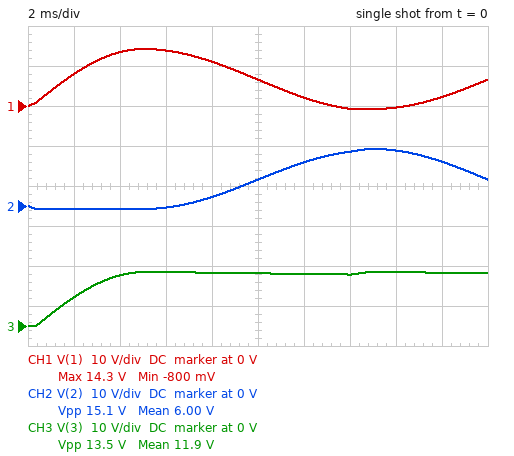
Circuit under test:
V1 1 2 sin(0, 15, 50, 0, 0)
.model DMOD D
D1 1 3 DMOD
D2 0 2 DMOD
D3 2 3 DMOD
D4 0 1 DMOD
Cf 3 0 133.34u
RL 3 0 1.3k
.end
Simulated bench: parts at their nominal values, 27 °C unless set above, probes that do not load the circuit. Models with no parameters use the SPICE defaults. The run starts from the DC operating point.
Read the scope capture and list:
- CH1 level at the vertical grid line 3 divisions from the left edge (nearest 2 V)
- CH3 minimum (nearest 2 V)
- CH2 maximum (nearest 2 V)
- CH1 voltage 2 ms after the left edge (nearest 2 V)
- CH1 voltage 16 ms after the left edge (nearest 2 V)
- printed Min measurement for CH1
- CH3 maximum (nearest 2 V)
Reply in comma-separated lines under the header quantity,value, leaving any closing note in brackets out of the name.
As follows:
quantity,value
CH1 level at the vertical grid line 3 divisions from the left edge,14 V
CH3 minimum,0 V
CH2 maximum,14 V
CH1 voltage 2 ms after the left edge,8 V
CH1 voltage 16 ms after the left edge,0 V
printed Min measurement for CH1,-800 mV
CH3 maximum,14 V
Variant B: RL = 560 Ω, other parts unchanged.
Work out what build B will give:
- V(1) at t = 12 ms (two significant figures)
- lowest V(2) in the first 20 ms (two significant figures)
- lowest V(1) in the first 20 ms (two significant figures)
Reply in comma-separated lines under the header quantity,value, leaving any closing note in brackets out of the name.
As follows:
quantity,value
V(1) at t = 12 ms,1.8 V
lowest V(2) in the first 20 ms,-820 mV
lowest V(1) in the first 20 ms,-800 mV
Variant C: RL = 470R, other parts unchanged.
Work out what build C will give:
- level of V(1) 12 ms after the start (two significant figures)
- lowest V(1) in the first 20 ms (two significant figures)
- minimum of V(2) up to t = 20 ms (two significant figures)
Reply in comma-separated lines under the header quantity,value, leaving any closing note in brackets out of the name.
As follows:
quantity,value
level of V(1) 12 ms after the start,1.7 V
lowest V(1) in the first 20 ms,-800 mV
minimum of V(2) up to t = 20 ms,-820 mV
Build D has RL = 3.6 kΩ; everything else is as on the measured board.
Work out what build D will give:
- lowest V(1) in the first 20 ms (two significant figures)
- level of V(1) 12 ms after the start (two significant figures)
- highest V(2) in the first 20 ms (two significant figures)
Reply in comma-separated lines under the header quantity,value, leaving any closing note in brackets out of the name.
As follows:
quantity,value
lowest V(1) in the first 20 ms,-770 mV
level of V(1) 12 ms after the start,2.3 V
highest V(2) in the first 20 ms,14 V
